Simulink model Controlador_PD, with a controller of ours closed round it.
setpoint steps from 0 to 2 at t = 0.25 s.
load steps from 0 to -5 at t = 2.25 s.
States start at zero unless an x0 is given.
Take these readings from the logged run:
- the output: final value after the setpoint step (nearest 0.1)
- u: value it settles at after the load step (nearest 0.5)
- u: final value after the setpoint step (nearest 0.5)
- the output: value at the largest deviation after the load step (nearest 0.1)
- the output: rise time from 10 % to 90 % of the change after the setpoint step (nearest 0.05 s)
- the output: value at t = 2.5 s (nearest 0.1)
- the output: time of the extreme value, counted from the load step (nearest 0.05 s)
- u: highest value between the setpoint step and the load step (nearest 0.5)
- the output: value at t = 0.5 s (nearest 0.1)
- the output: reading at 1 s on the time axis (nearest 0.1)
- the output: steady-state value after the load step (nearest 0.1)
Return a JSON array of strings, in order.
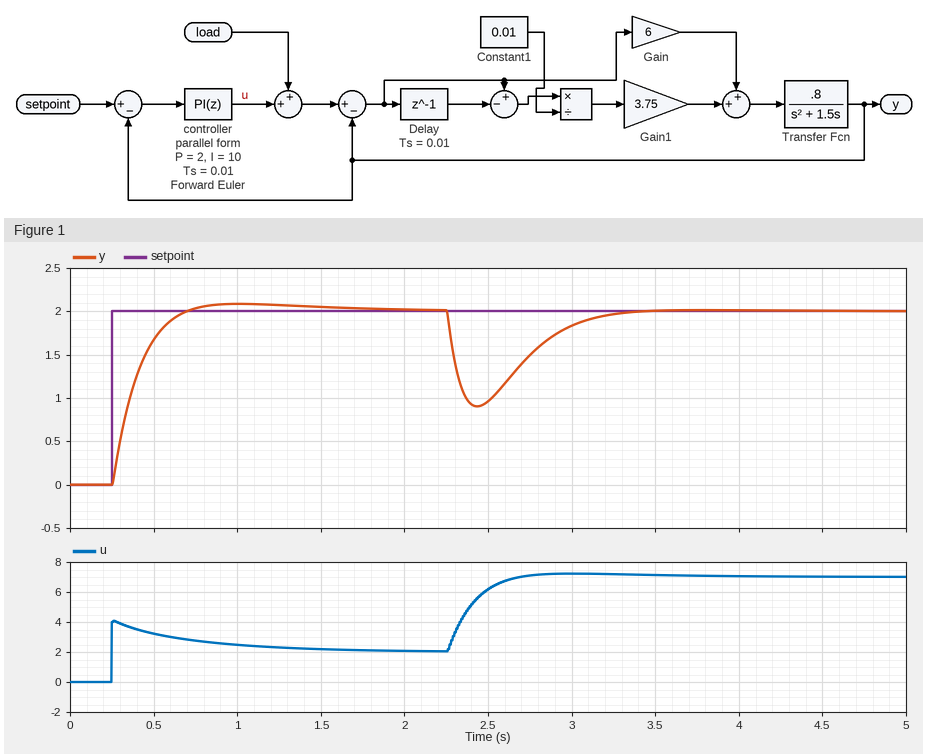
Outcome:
["2.0", "7.0", "2.0", "0.9", "0.30 s", "1.0", "0.20 s", "4.0", "1.7", "2.1", "2.0"]
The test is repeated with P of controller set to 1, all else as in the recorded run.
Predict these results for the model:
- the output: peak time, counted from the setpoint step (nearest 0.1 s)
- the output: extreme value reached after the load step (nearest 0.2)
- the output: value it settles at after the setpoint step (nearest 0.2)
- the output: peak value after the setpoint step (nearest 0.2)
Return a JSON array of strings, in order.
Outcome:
["0.6 s", "0.6", "2.0", "2.2"]
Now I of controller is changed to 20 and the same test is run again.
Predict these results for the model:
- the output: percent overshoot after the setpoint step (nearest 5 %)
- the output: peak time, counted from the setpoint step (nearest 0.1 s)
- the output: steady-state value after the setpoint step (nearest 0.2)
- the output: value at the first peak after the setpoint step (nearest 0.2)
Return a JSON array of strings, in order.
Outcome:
["15 %", "0.4 s", "2.0", "2.2"]
